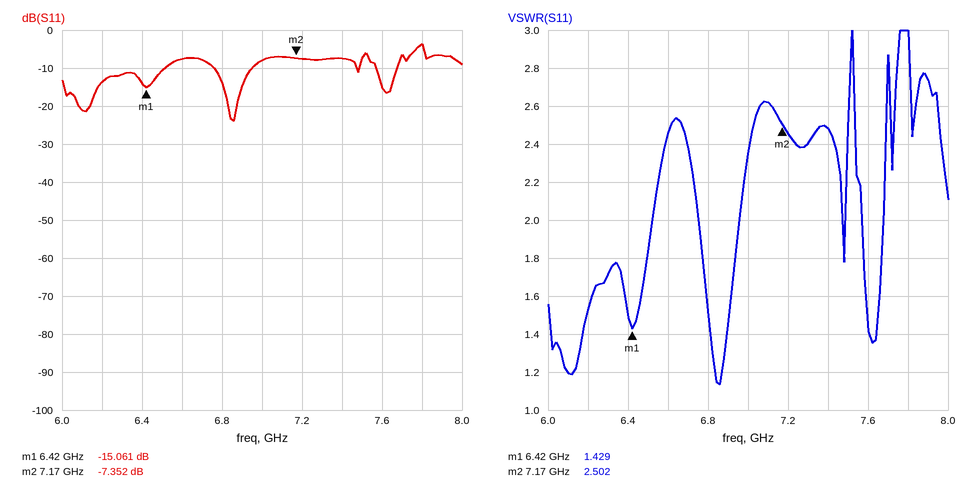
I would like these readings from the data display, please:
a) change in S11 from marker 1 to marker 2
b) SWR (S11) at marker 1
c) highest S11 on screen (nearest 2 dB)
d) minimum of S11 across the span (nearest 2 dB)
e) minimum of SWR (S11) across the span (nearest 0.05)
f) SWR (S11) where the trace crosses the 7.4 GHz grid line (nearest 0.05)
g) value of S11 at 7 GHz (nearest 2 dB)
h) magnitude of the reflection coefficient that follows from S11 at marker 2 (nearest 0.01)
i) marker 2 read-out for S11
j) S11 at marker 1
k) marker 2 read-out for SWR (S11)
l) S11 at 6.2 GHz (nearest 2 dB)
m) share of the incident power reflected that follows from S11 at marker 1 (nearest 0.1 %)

7.709 dB
1.429
-4 dB
-24 dB
1.15
2.50
-8 dB
0.43
-7.352 dB
-15.061 dB
2.502
-14 dB
3.1 %
